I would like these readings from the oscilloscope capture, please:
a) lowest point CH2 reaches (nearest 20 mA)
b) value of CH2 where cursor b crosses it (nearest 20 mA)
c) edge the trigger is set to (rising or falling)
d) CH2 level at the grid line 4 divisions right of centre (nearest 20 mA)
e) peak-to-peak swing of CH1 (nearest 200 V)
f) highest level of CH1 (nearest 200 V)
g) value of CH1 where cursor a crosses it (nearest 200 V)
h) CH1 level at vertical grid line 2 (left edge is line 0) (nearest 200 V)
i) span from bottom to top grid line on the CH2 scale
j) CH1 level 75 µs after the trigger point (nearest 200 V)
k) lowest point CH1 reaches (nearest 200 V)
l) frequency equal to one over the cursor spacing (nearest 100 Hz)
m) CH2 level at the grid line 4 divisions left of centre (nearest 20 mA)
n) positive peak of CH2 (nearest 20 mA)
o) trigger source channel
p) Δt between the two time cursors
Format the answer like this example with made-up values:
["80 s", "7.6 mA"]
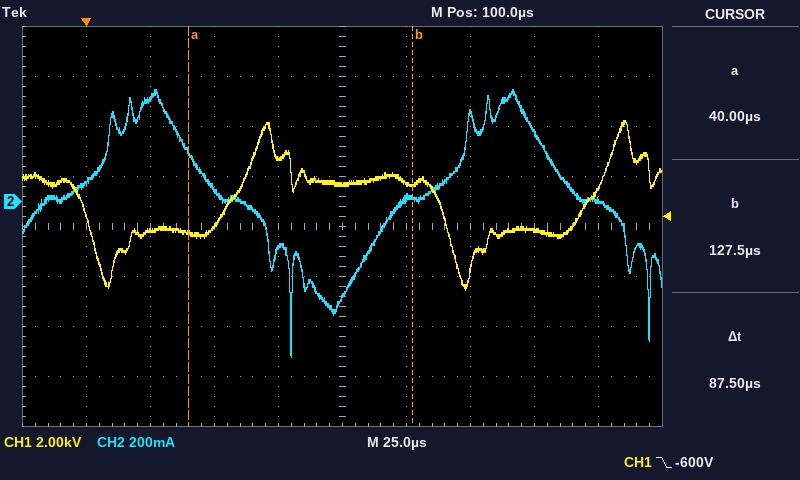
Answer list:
["-620 mA", "20 mA", "falling", "0 mA", "6.8 kV", "3.2 kV", "-1.2 kV", "-1.2 kV", "1.6 A", "1.8 kV", "-3.6 kV", "11.4 kHz", "80 mA", "440 mA", "CH1", "87.5 µs"]
